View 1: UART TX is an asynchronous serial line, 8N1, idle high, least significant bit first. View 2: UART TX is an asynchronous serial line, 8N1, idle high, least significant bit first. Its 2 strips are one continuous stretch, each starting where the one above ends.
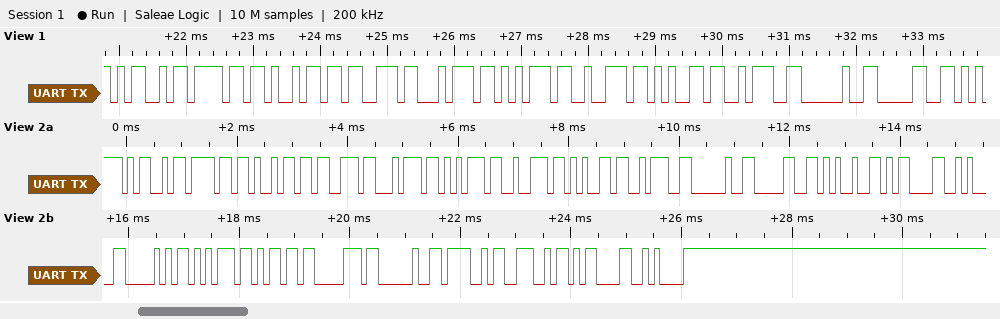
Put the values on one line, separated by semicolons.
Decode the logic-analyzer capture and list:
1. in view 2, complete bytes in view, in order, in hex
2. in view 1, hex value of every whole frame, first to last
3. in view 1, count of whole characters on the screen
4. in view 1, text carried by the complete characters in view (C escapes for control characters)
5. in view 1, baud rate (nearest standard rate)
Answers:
4D 6F 69 73 74 75 72 65 3A 20 30 25 0D 0A 50 75 6D 70 20 4F 4E 0D 0A; 4D 6F 69 73 74 75 72 65 3A 20 30; 11; "Moisture: 0"; 9600 baud
